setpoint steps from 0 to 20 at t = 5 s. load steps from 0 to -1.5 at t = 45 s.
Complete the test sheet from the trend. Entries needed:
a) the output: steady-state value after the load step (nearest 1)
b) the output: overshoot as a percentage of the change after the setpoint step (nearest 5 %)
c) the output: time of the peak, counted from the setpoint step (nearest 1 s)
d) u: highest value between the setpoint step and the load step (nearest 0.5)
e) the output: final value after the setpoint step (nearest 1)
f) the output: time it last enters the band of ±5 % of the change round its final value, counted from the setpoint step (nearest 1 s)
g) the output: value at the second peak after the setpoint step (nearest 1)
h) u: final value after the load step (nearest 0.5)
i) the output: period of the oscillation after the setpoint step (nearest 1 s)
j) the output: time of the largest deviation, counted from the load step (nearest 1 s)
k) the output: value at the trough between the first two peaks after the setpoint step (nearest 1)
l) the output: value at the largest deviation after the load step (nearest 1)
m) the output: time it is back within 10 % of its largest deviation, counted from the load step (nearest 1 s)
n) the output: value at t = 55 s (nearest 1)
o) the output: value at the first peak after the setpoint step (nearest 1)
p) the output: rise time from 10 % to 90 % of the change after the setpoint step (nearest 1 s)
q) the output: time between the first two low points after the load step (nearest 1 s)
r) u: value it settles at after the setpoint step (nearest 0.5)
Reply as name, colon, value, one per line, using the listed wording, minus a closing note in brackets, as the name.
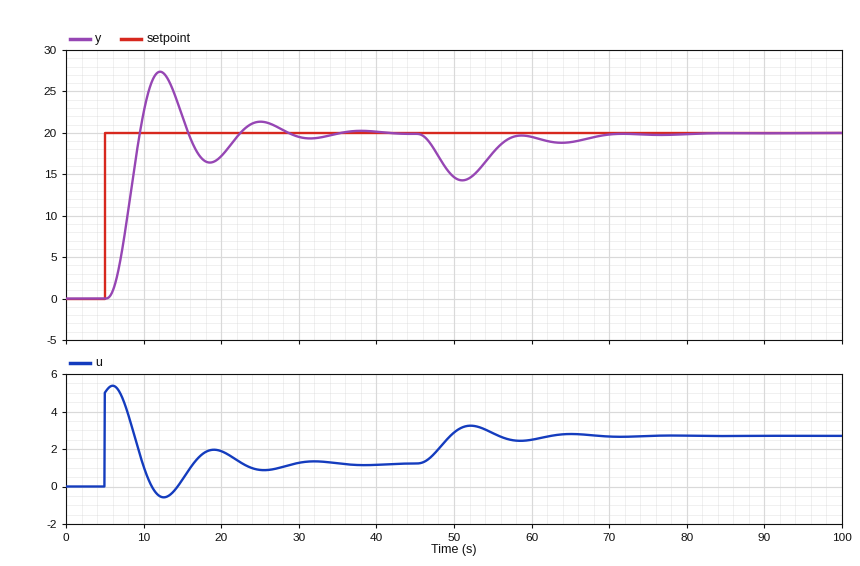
the output: steady-state value after the load step: 20
the output: overshoot as a percentage of the change after the setpoint step: 35 %
the output: time of the peak, counted from the setpoint step: 7 s
u: highest value between the setpoint step and the load step: 5.5
the output: final value after the setpoint step: 20
the output: time it last enters the band of ±5 % of the change round its final value, counted from the setpoint step: 22 s
the output: value at the second peak after the setpoint step: 21
u: final value after the load step: 2.5
the output: period of the oscillation after the setpoint step: 13 s
the output: time of the largest deviation, counted from the load step: 6 s
the output: value at the trough between the first two peaks after the setpoint step: 16
the output: value at the largest deviation after the load step: 14
the output: time it is back within 10 % of its largest deviation, counted from the load step: 23 s
the output: value at t = 55 s: 18
the output: value at the first peak after the setpoint step: 27
the output: rise time from 10 % to 90 % of the change after the setpoint step: 3 s
the output: time between the first two low points after the load step: 13 s
u: value it settles at after the setpoint step: 1.0
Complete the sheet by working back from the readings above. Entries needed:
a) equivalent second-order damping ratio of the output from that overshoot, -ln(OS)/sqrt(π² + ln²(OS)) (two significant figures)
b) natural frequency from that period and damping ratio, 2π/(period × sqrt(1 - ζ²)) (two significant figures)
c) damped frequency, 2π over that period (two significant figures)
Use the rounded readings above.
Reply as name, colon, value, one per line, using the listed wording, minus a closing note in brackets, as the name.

equivalent second-order damping ratio of the output from that overshoot, -ln(OS)/sqrt(π² + ln²(OS)): 0.32
natural frequency from that period and damping ratio, 2π/(period × sqrt(1 - ζ²)): 0.51 rad/s
damped frequency, 2π over that period: 0.48 rad/s
